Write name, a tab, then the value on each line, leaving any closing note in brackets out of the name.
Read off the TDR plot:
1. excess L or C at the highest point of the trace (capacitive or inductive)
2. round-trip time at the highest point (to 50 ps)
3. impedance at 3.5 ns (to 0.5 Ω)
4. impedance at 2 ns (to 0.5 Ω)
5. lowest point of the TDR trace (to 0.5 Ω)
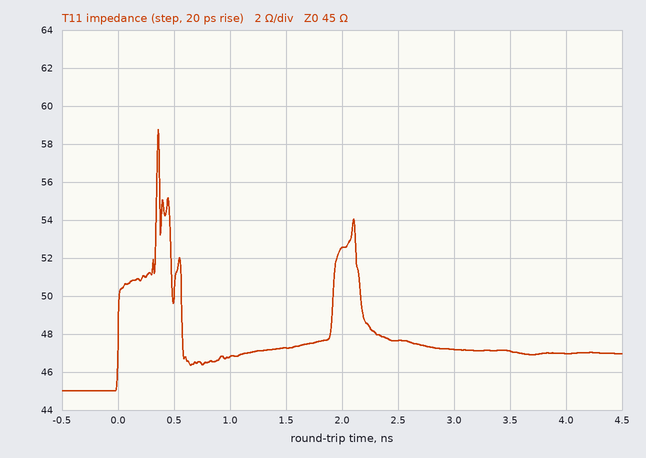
excess L or C at the highest point of the trace	inductive
round-trip time at the highest point	350 ps
impedance at 3.5 ns	47.0 Ω
impedance at 2 ns	52.5 Ω
lowest point of the TDR trace	45.0 Ω
